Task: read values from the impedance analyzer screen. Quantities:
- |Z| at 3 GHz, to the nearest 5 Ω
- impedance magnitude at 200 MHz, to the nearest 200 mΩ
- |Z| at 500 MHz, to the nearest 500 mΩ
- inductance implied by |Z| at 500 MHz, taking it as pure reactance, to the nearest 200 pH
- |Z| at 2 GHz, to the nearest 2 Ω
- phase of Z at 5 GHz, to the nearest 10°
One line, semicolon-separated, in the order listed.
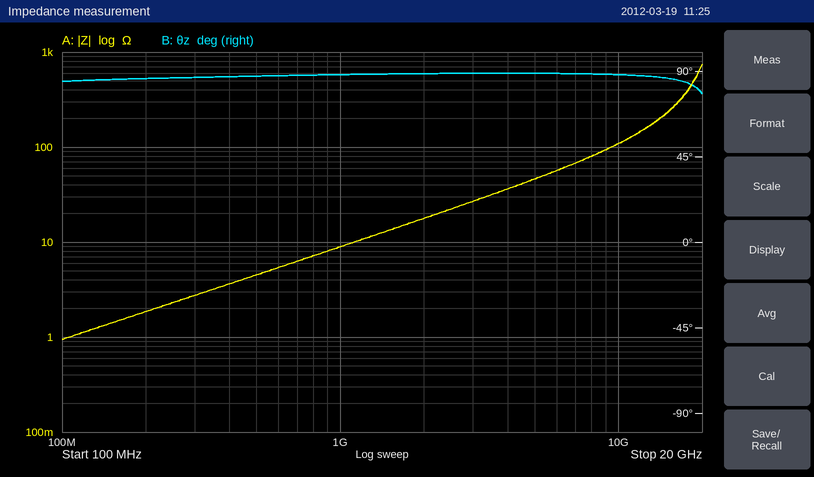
25 Ω; 1.8 Ω; 4.5 Ω; 1.4 nH; 18 Ω; 90°
